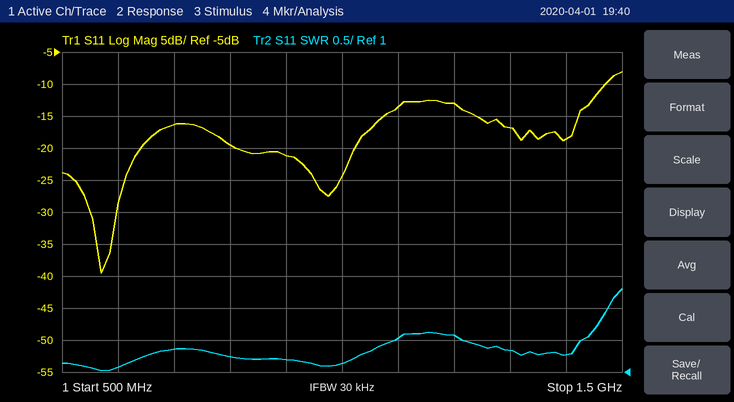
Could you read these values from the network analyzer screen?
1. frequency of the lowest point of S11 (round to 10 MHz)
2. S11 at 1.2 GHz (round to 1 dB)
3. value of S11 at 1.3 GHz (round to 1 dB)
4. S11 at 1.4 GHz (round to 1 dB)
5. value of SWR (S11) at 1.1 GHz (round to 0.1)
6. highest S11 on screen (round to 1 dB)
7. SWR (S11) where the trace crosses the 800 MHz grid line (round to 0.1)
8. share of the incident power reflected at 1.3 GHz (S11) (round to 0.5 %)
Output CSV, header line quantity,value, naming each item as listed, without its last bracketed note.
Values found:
quantity,value
frequency of the lowest point of S11,570 MHz
S11 at 1.2 GHz,-13 dB
value of S11 at 1.3 GHz,-17 dB
S11 at 1.4 GHz,-19 dB
value of SWR (S11) at 1.1 GHz,1.5
highest S11 on screen,-8 dB
SWR (S11) where the trace crosses the 800 MHz grid line,1.2
share of the incident power reflected at 1.3 GHz (S11),2.0 %
